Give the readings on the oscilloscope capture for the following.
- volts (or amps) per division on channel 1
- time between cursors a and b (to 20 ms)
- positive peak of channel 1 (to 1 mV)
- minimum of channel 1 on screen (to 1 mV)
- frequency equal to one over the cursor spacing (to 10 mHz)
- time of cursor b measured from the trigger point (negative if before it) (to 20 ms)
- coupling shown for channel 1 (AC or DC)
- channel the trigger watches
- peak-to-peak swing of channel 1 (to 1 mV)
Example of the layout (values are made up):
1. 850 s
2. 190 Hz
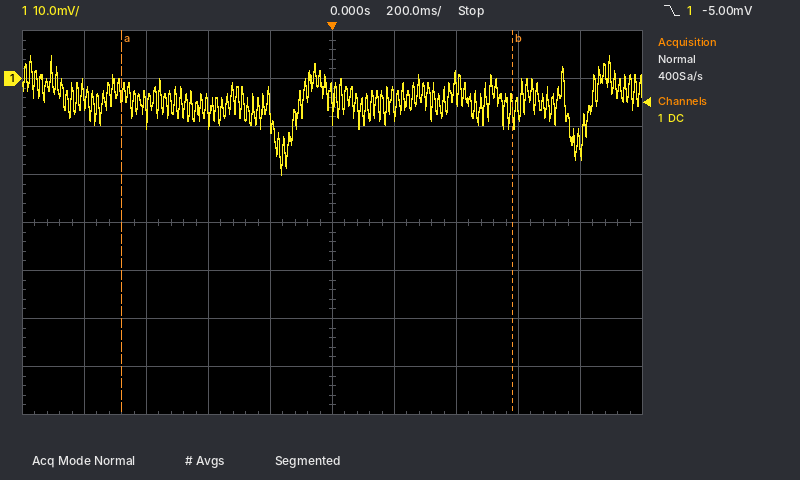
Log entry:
1. 10 mV
2. 1.26 s
3. 5 mV
4. -20 mV
5. 790 mHz
6. +580 ms
7. DC
8. channel 1
9. 25 mV
